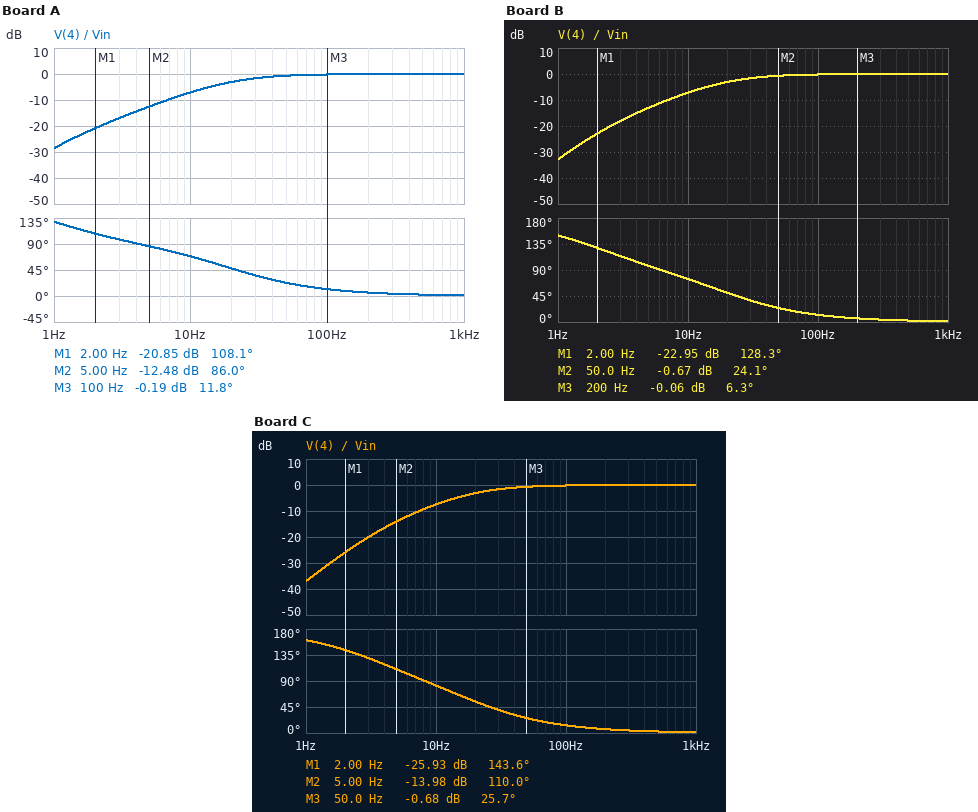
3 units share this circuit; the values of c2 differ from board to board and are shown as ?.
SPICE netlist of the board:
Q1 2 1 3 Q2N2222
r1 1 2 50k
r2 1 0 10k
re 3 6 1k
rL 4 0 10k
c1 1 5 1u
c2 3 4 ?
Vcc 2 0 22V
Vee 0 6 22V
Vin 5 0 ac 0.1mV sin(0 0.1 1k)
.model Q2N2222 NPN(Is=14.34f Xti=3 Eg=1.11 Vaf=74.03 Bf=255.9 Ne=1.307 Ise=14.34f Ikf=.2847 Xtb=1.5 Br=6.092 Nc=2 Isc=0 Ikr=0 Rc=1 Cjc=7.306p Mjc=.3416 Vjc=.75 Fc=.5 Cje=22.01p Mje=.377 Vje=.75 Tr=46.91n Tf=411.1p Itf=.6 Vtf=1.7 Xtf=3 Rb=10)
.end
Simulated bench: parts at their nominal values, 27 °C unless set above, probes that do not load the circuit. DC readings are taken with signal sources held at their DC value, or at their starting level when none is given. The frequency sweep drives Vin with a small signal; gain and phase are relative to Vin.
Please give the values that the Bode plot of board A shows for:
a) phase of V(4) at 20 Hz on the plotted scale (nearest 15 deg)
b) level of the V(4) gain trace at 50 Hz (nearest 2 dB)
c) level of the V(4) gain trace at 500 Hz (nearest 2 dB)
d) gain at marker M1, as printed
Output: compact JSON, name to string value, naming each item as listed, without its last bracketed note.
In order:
{"phase of V(4) at 20 Hz on the plotted scale": "45 deg", "level of the V(4) gain trace at 50 Hz": "0 dB", "level of the V(4) gain trace at 500 Hz": "0 dB", "gain at marker M1, as printed": "-20.85 dB"}
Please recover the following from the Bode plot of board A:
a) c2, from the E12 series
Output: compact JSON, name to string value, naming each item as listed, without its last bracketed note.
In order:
{"c2, from the E12 series": "18 µF"}
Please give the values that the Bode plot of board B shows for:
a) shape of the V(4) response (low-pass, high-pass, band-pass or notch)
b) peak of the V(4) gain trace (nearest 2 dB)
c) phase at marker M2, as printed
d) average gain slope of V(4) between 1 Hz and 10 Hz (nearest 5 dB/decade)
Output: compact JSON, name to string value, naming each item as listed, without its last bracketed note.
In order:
{"shape of the V(4) response": "high-pass", "peak of the V(4) gain trace": "0 dB", "phase at marker M2, as printed": "24.1 deg", "average gain slope of V(4) between 1 Hz and 10 Hz": "25 dB/decade"}
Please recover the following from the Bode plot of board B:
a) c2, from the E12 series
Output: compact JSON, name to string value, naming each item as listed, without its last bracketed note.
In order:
{"c2, from the E12 series": "8.2 µF"}
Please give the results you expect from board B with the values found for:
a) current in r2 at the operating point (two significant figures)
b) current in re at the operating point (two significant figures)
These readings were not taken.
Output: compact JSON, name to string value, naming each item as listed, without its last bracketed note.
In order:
{"current in r2 at the operating point": "280 µA", "current in re at the operating point": "24 mA"}
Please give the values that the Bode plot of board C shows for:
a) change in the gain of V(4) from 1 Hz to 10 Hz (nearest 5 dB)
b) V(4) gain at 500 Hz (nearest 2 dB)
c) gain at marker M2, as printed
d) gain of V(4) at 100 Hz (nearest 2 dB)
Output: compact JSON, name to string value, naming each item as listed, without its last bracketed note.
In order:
{"change in the gain of V(4) from 1 Hz to 10 Hz": "30 dB", "V(4) gain at 500 Hz": "0 dB", "gain at marker M2, as printed": "-13.98 dB", "gain of V(4) at 100 Hz": "0 dB"}
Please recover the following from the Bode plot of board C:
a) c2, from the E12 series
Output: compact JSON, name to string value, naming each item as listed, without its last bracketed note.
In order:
{"c2, from the E12 series": "4.7 µF"}
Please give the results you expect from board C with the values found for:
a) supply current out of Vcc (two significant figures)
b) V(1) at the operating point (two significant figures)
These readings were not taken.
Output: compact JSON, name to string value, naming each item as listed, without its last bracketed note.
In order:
{"supply current out of Vcc": "24 mA", "V(1) at the operating point": "2.8 V"}
